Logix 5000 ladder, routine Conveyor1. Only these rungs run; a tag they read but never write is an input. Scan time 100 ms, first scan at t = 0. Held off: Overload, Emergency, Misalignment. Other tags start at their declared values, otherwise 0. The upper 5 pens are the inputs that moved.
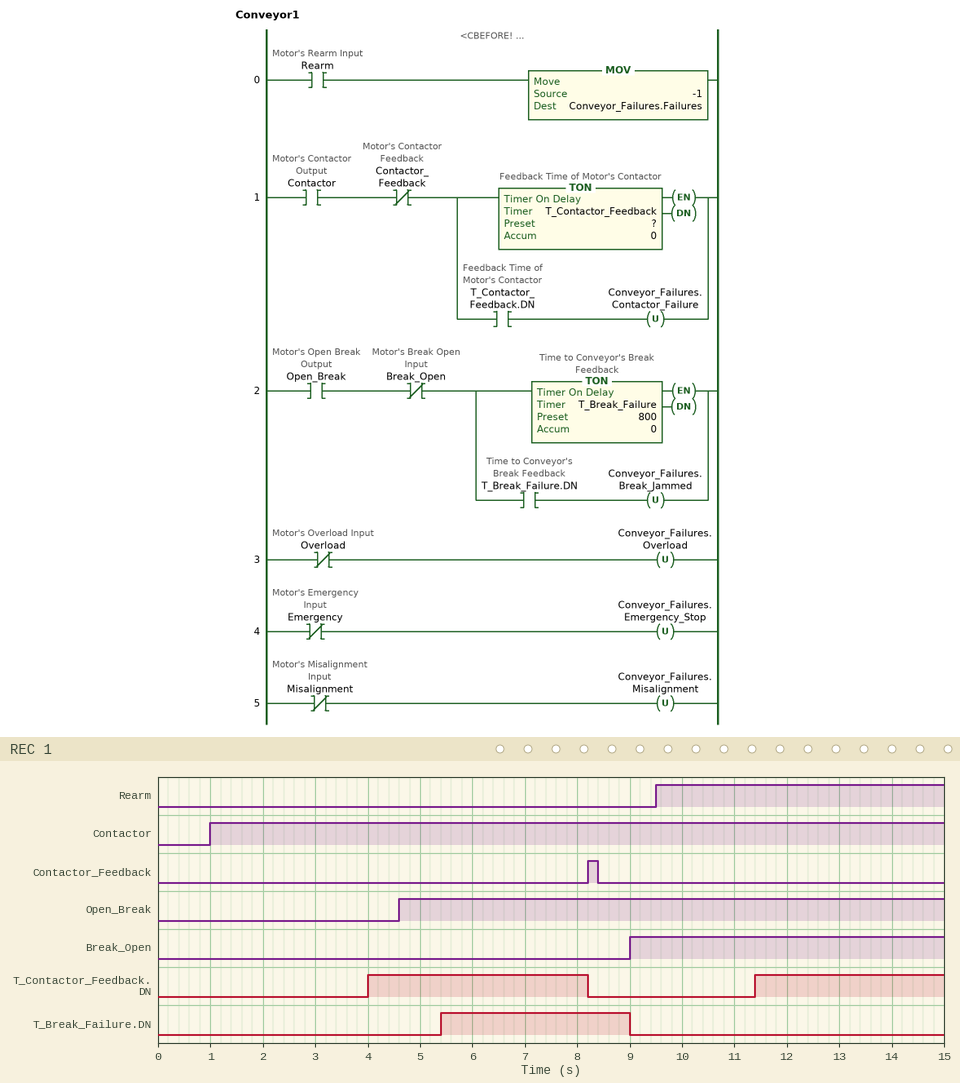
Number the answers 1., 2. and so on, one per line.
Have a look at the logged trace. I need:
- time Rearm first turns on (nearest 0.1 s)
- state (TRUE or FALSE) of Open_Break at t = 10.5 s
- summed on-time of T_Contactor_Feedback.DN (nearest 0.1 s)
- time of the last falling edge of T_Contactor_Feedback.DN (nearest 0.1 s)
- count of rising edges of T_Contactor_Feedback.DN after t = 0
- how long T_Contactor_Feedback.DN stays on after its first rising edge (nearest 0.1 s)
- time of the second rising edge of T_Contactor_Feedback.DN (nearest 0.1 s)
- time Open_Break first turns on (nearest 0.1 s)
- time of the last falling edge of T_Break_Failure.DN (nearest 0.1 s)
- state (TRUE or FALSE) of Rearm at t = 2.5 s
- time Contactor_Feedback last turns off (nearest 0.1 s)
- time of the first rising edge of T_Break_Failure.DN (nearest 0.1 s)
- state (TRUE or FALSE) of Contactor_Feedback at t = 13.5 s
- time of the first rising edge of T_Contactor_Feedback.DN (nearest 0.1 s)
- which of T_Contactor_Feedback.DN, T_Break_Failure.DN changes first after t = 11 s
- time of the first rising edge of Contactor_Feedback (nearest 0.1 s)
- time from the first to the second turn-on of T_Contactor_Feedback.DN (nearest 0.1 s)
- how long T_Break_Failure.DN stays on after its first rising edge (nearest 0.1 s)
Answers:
1. 9.5 s
2. TRUE
3. 7.8 s
4. 8.2 s
5. 2
6. 4.2 s
7. 11.4 s
8. 4.6 s
9. 9.0 s
10. FALSE
11. 8.4 s
12. 5.4 s
13. FALSE
14. 4.0 s
15. T_Contactor_Feedback.DN
16. 8.2 s
17. 7.4 s
18. 3.6 s
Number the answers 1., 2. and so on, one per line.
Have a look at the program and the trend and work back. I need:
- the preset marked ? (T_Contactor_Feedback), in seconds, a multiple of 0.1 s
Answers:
1. 3.0 s
